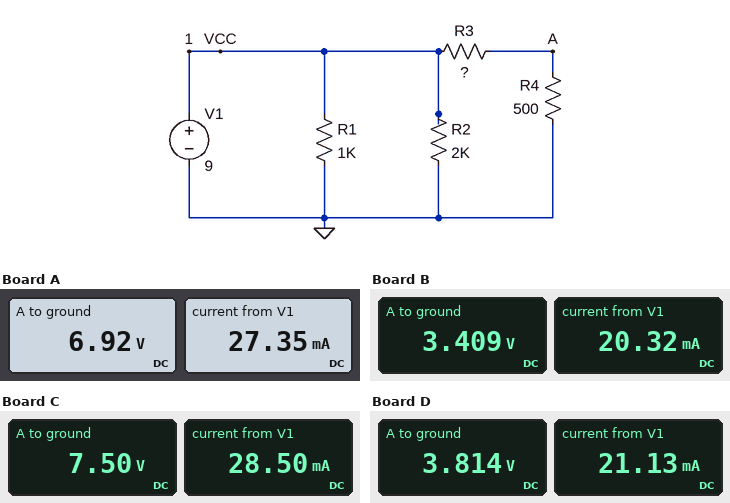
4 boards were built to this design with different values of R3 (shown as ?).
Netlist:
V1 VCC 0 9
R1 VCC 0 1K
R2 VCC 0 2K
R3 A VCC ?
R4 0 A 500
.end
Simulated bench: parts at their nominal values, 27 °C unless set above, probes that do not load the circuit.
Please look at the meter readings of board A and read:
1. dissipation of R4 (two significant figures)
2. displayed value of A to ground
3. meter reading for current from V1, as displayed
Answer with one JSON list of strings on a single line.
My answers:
["96 mW", "6.92 V", "27.35 mA"]
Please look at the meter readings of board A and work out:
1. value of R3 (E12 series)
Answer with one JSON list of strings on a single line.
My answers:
["150 Ω"]
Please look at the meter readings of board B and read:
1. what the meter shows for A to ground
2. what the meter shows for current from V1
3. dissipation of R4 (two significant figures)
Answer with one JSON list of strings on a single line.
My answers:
["3.409 V", "20.32 mA", "23 mW"]
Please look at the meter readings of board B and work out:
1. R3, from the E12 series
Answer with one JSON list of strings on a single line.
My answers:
["820 Ω"]
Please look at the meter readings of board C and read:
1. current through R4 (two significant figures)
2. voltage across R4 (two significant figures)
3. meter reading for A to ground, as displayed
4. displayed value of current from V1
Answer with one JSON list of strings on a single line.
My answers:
["15 mA", "7.5 V", "7.50 V", "28.50 mA"]
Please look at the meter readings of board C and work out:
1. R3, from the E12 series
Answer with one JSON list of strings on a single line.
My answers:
["100 Ω"]
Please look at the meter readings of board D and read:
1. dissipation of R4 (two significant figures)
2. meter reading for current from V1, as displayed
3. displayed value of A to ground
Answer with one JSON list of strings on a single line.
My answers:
["29 mW", "21.13 mA", "3.814 V"]
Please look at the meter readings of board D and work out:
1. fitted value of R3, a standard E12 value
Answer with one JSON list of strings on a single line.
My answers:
["680 Ω"]
